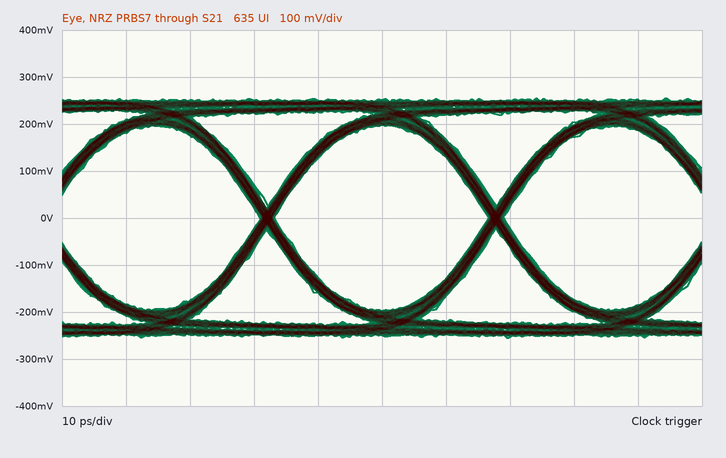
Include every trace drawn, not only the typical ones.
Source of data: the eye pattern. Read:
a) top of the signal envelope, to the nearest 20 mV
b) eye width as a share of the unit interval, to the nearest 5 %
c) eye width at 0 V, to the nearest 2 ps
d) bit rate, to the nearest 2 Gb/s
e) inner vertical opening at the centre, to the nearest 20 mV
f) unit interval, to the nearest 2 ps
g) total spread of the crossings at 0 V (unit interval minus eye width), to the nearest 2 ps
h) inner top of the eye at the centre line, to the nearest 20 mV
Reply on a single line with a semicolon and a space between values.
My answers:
260 mV; 95 %; 34 ps; 28 Gb/s; 400 mV; 36 ps; 2 ps; 200 mV
